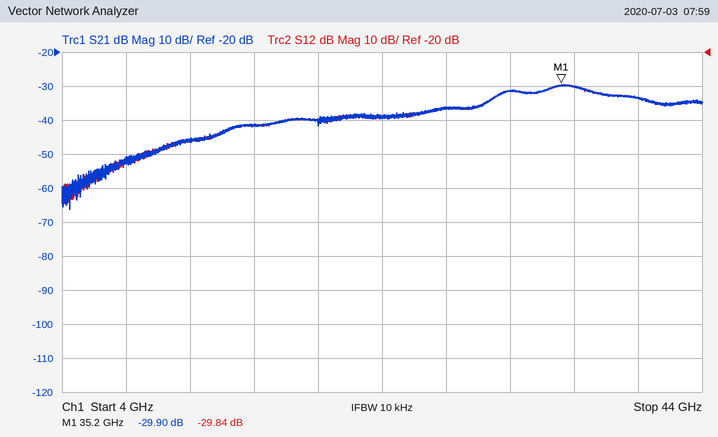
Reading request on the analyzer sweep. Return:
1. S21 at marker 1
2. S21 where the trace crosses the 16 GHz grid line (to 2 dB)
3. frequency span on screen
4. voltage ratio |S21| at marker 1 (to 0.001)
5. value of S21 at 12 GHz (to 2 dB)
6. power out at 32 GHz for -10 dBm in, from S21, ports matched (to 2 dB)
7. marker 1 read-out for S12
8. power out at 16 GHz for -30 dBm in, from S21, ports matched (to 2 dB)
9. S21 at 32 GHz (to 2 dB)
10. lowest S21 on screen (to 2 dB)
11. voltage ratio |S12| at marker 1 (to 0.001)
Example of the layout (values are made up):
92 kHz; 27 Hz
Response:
-29.90 dB; -42 dB; 40 GHz; 0.032; -46 dB; -42 dBm; -29.84 dB; -72 dBm; -32 dB; -66 dB; 0.032
